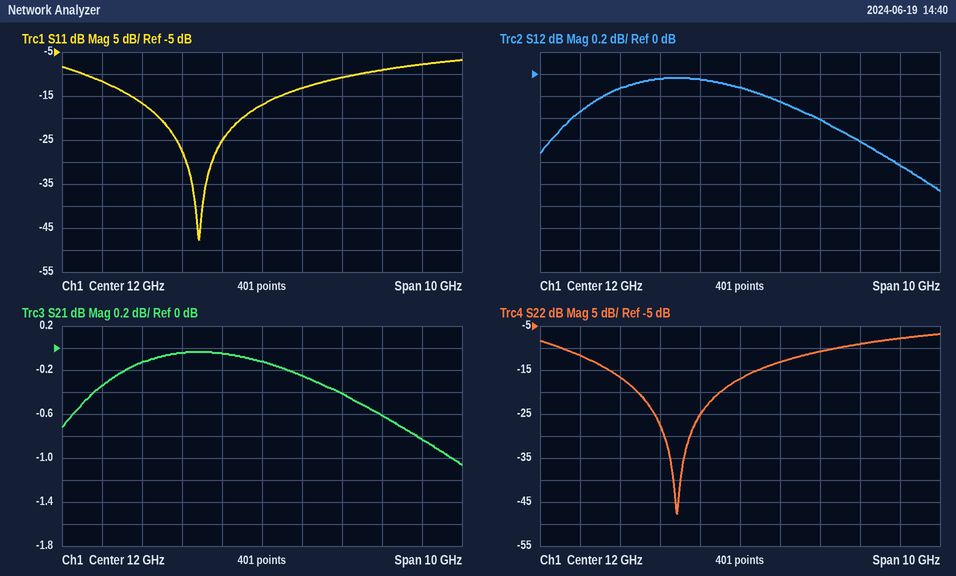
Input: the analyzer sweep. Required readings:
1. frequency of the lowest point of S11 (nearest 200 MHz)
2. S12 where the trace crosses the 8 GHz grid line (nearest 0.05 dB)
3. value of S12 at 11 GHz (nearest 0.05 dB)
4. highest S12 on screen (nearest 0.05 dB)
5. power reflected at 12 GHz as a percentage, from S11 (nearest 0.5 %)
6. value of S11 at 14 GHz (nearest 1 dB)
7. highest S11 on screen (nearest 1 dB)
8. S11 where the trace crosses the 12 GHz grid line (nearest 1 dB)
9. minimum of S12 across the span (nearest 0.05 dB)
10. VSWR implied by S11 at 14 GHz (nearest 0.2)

10.4 GHz
-0.35 dB
-0.05 dB
-0.05 dB
2.0 %
-11 dB
-7 dB
-17 dB
-1.05 dB
1.8
